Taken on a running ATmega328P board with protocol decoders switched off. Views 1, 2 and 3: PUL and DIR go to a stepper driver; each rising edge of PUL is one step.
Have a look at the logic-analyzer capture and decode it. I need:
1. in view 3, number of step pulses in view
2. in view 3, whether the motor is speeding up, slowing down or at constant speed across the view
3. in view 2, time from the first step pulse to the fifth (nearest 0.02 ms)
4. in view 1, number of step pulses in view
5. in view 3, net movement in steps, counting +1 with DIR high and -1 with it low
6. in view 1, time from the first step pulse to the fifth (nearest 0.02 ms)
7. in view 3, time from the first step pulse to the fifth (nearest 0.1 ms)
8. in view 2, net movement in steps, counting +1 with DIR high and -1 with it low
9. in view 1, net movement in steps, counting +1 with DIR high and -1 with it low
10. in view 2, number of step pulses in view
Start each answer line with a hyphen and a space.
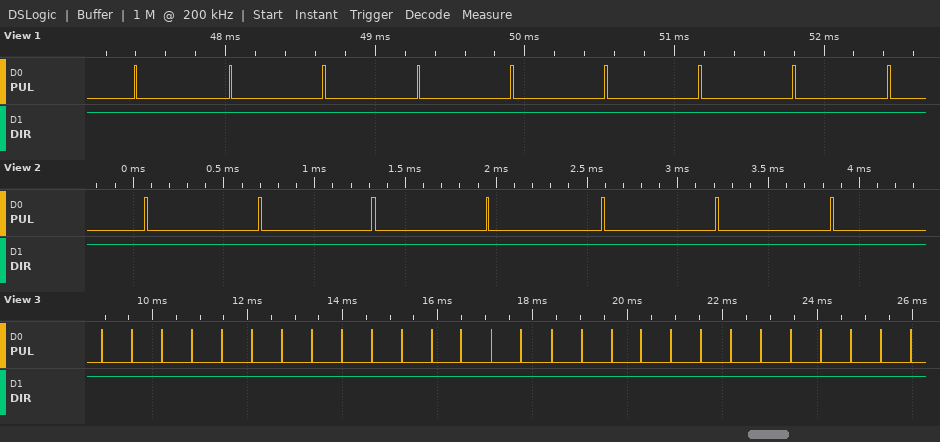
- 28
- constant speed
- 2.52 ms
- 9
- +28
- 2.52 ms
- 2.5 ms
- +7
- +9
- 7
